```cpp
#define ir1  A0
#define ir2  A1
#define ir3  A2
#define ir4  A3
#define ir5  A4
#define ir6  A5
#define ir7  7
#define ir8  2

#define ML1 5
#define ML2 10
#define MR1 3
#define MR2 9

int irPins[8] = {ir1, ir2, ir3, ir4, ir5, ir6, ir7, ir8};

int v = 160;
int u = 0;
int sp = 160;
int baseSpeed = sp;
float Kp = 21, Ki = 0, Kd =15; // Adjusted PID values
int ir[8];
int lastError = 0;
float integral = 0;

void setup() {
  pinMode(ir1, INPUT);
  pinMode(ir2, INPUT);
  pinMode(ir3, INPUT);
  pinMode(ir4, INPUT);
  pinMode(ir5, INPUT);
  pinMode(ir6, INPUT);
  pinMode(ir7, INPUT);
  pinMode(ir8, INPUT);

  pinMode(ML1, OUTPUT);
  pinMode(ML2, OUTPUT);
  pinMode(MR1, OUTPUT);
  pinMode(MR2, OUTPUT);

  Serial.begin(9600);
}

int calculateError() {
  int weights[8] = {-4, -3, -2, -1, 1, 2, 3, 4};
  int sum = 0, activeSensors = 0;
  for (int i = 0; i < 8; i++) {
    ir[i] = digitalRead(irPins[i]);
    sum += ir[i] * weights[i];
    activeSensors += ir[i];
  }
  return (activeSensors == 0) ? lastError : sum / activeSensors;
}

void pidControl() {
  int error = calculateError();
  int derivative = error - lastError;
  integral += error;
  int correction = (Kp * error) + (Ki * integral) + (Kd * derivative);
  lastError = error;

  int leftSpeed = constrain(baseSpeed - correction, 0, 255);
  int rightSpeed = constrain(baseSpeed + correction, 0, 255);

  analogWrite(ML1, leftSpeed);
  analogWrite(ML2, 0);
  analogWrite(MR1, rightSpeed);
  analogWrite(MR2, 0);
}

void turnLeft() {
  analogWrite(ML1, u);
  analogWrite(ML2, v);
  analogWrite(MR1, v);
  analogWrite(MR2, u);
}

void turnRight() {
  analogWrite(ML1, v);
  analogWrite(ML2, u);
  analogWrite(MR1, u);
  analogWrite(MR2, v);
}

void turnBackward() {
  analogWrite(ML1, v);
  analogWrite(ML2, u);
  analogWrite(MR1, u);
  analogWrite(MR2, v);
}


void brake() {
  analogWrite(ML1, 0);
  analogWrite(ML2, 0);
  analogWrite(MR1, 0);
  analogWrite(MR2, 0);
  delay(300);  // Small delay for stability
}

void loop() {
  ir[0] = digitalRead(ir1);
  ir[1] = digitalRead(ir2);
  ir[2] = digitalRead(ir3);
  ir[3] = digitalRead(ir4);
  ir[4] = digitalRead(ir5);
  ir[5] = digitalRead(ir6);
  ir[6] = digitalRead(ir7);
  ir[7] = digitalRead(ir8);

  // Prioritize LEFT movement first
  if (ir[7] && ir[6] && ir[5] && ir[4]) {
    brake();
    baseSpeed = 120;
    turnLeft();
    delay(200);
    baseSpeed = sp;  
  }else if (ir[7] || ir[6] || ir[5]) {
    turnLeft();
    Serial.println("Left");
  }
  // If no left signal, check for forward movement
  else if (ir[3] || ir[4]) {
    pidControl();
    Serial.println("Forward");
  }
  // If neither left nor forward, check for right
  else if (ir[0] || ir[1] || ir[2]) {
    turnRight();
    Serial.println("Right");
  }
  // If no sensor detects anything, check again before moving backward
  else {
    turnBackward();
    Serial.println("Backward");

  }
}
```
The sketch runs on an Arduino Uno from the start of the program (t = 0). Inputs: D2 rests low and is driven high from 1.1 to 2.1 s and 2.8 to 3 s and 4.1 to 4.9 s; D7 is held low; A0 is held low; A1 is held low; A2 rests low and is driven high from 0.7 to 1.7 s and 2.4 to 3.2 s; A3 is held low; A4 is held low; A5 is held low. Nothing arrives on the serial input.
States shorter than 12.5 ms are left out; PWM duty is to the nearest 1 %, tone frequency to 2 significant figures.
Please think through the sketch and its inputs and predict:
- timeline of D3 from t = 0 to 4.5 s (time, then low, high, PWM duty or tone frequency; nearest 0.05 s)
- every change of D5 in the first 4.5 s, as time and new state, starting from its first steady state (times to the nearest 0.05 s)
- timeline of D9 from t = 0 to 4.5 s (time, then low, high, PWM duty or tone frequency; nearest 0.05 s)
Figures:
0 s low; 1.1 s PWM 63 %; 2.1 s low; 2.8 s PWM 63 %; 3 s low; 4.1 s PWM 63 %
0 s PWM 63 %; 1.1 s low; 2.1 s PWM 63 %; 2.8 s low; 3 s PWM 63 %; 4.1 s low
0 s PWM 63 %; 1.1 s low; 2.1 s PWM 63 %; 2.8 s low; 3 s PWM 63 %; 4.1 s low
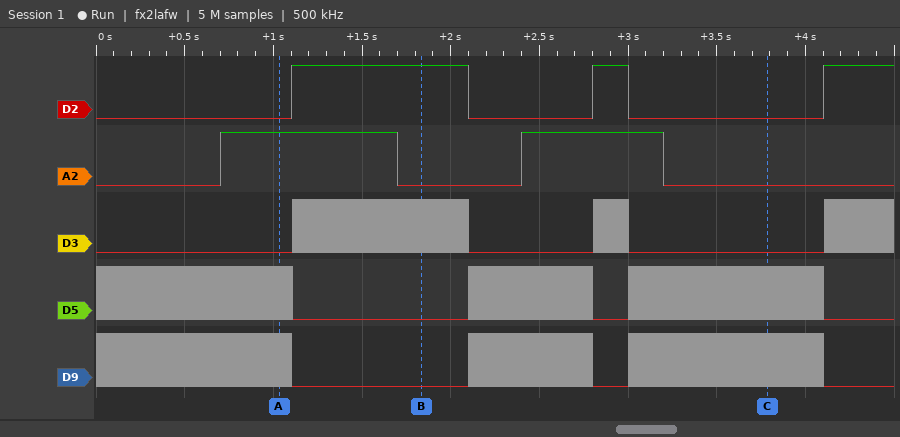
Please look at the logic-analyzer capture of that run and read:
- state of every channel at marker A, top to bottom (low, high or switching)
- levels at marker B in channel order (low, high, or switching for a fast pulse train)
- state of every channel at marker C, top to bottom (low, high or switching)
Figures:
D2 low, A2 high, D3 low, D5 switching, D9 switching
D2 high, A2 low, D3 switching, D5 low, D9 low
D2 low, A2 low, D3 low, D5 switching, D9 switching
